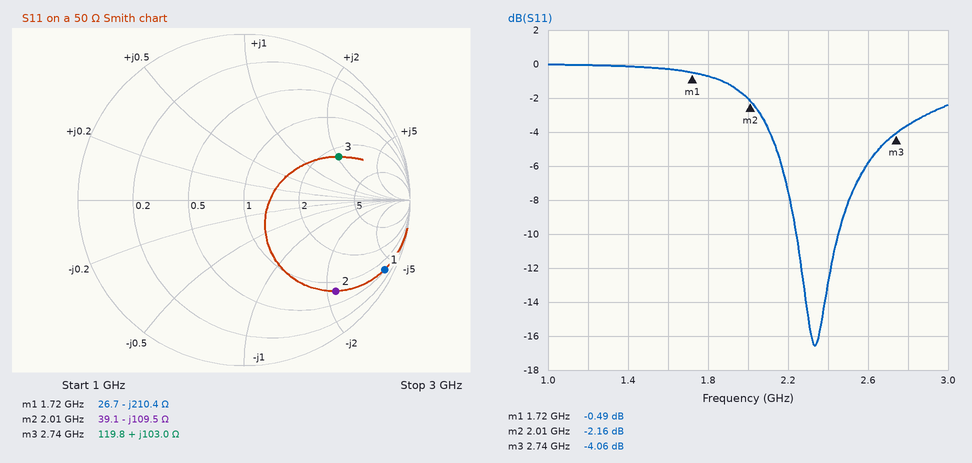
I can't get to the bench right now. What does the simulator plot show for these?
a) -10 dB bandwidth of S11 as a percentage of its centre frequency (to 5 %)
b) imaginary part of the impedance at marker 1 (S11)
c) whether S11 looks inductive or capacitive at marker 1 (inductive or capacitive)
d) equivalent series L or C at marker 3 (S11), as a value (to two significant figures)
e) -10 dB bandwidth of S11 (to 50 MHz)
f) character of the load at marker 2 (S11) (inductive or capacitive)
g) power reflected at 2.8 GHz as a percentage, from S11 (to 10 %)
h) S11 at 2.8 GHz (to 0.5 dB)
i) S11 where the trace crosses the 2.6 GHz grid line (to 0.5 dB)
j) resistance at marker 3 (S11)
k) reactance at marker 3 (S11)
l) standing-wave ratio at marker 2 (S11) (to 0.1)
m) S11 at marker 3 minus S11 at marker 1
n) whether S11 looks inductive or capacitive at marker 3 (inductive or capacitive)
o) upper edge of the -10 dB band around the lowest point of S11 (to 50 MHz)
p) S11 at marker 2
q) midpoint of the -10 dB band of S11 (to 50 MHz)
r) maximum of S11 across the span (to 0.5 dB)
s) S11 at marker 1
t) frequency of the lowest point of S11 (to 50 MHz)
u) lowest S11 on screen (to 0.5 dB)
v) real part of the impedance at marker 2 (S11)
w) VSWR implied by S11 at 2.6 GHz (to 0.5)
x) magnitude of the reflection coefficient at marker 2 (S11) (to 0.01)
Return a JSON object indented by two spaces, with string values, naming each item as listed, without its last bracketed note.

{
  "-10 dB bandwidth of S11 as a percentage of its centre frequency": "10 %",
  "imaginary part of the impedance at marker 1": "-210.4 Ω",
  "whether S11 looks inductive or capacitive at marker 1": "capacitive",
  "equivalent series L or C at marker 3 (S11), as a value": "6.0 nH",
  "-10 dB bandwidth of S11": "200 MHz",
  "character of the load at marker 2 (S11)": "capacitive",
  "power reflected at 2.8 GHz as a percentage, from S11": "40 %",
  "S11 at 2.8 GHz": "-3.5 dB",
  "S11 where the trace crosses the 2.6 GHz grid line": "-6.0 dB",
  "resistance at marker 3": "119.8 Ω",
  "reactance at marker 3": "+103.0 Ω",
  "standing-wave ratio at marker 2 (S11)": "8.1",
  "S11 at marker 3 minus S11 at marker 1": "-3.57 dB",
  "whether S11 looks inductive or capacitive at marker 3": "inductive",
  "upper edge of the -10 dB band around the lowest point of S11": "2.45 GHz",
  "S11 at marker 2": "-2.16 dB",
  "midpoint of the -10 dB band of S11": "2.35 GHz",
  "maximum of S11 across the span": "0.0 dB",
  "S11 at marker 1": "-0.49 dB",
  "frequency of the lowest point of S11": "2.35 GHz",
  "lowest S11 on screen": "-16.5 dB",
  "real part of the impedance at marker 2": "39.1 Ω",
  "VSWR implied by S11 at 2.6 GHz": "3.0",
  "magnitude of the reflection coefficient at marker 2 (S11)": "0.78"
}
